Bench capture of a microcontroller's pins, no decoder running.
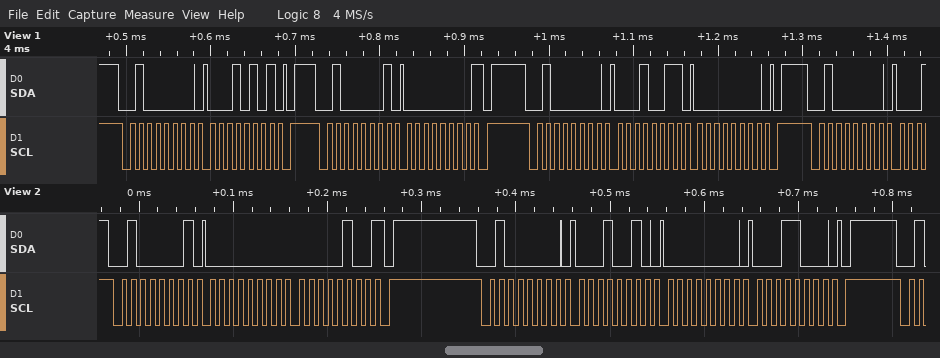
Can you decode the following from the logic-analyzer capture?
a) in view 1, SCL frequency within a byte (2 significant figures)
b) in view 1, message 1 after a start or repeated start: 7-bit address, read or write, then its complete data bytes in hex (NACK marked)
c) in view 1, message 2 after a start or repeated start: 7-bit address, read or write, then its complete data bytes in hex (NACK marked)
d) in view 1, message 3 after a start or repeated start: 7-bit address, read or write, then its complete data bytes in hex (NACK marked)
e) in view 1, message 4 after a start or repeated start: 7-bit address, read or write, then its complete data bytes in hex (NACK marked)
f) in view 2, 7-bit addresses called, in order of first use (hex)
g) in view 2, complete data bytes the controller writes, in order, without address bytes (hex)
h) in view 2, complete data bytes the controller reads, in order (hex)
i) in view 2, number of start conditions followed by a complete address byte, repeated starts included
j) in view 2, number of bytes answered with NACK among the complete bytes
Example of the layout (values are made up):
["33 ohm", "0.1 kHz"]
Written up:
["100 kHz", "0x20 write: 15", "0x20 read: 00 NACK", "0x20 write: 13 00", "0x20 write", "0x20", "12 00 18", "00 04", "2", "1"]
